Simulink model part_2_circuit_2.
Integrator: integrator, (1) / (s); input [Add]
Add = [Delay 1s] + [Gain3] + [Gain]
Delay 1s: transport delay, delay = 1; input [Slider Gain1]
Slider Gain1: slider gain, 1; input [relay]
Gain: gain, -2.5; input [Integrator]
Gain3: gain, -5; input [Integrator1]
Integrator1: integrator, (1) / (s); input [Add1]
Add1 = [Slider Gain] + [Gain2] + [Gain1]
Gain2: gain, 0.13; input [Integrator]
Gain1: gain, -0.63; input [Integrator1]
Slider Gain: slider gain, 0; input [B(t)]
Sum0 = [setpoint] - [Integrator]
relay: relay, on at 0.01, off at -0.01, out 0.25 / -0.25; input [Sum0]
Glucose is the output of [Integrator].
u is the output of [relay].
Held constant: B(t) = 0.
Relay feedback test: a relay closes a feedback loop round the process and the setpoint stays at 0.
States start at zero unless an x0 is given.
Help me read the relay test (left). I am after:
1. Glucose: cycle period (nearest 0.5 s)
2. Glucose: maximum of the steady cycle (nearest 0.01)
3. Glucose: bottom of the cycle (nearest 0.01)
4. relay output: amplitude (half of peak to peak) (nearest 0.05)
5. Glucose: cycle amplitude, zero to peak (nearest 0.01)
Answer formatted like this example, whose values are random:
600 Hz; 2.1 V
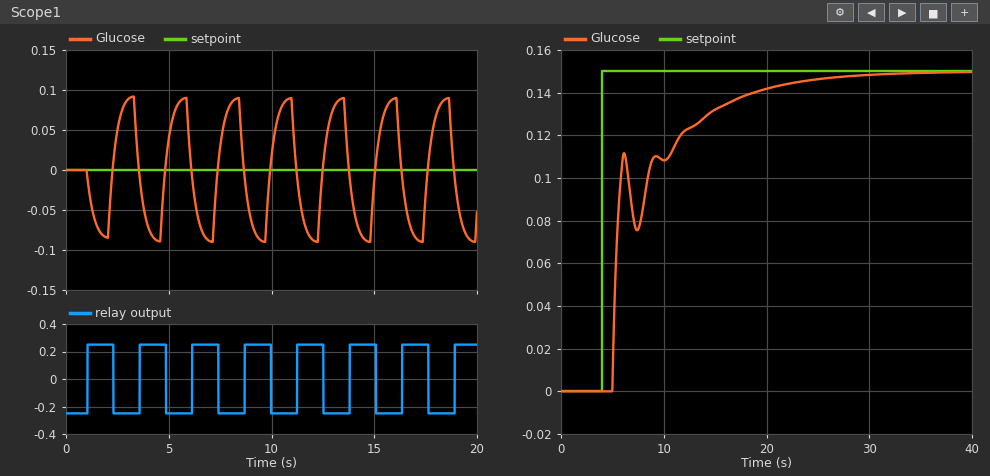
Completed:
2.5 s; 0.09; -0.09; 0.25; 0.09
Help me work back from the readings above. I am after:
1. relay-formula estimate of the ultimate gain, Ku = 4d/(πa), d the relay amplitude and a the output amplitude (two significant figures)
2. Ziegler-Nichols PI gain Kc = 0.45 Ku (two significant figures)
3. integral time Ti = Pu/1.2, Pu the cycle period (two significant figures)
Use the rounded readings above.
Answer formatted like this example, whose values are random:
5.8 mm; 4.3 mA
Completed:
3.5; 1.6; 2.1 s
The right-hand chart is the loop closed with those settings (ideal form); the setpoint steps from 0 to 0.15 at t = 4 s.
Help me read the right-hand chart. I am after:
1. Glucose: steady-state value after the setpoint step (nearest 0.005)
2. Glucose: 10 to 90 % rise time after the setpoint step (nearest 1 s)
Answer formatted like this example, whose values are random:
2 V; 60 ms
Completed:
0.150; 11 s
